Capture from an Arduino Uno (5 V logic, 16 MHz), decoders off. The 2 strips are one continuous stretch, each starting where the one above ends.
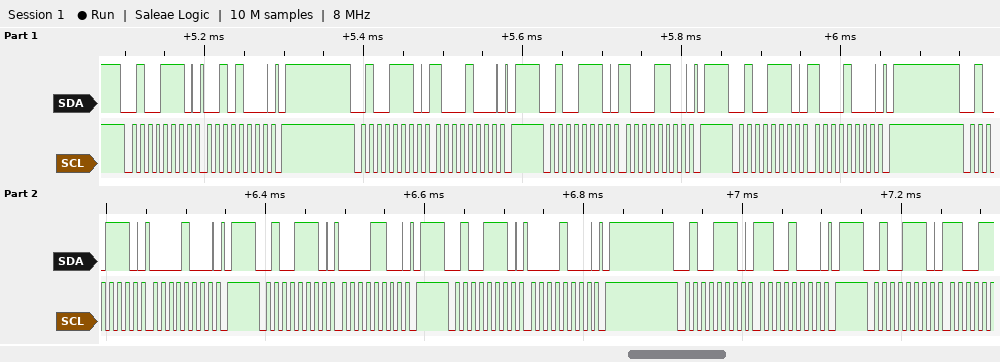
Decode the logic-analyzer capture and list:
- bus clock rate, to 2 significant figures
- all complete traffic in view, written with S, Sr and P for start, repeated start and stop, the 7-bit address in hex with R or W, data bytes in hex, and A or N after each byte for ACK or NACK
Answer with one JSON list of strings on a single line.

["100 kHz", "S 27W A 28 A P S 27W A 88 A P S 27W A 8C A P S 27W A 88 A P S 27W A 08 A P S 27W A 0C A P S 27W A 08 A P S 27W A C8 A P S 27W A"]
